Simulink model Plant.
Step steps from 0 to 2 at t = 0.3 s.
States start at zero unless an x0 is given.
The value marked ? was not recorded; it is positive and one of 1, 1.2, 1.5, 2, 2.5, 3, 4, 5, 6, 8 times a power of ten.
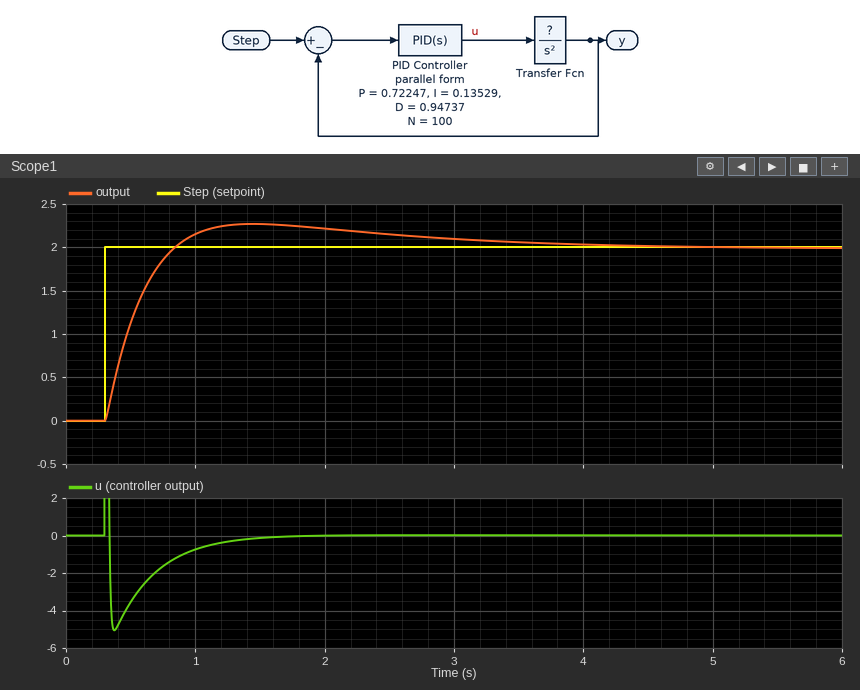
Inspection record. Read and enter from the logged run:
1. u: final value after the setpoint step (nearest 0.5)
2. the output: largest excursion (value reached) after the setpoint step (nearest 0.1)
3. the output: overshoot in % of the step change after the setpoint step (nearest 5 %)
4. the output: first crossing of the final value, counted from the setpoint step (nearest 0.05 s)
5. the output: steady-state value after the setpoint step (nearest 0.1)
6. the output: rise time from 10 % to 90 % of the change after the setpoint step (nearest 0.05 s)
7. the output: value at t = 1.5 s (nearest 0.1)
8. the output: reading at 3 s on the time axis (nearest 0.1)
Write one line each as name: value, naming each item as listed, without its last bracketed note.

u: final value after the setpoint step: 0.0
the output: largest excursion (value reached) after the setpoint step: 2.3
the output: overshoot in % of the step change after the setpoint step: 15 %
the output: first crossing of the final value, counted from the setpoint step: 0.55 s
the output: steady-state value after the setpoint step: 2.0
the output: rise time from 10 % to 90 % of the change after the setpoint step: 0.40 s
the output: value at t = 1.5 s: 2.3
the output: reading at 3 s on the time axis: 2.1
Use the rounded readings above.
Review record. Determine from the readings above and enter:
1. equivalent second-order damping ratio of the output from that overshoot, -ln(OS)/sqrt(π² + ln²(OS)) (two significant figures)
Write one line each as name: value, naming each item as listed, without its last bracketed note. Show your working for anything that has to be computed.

equivalent second-order damping ratio of the output from that overshoot, -ln(OS)/sqrt(π² + ln²(OS)): ln(0.15) = -1.897; 1.897 / sqrt(9.870 + 3.599) = 0.52
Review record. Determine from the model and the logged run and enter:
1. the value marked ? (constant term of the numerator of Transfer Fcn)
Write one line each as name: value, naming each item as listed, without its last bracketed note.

the value marked ?: 4
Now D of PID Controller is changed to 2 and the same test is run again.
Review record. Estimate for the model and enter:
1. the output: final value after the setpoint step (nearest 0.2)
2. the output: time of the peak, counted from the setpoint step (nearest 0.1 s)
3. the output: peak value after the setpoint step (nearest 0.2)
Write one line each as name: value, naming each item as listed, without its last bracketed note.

the output: final value after the setpoint step: 2.0
the output: time of the peak, counted from the setpoint step: 0.8 s
the output: peak value after the setpoint step: 2.0
